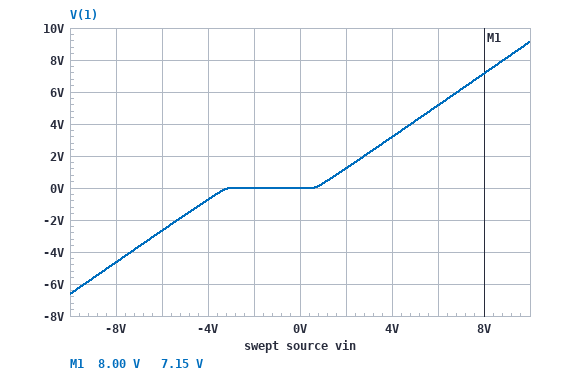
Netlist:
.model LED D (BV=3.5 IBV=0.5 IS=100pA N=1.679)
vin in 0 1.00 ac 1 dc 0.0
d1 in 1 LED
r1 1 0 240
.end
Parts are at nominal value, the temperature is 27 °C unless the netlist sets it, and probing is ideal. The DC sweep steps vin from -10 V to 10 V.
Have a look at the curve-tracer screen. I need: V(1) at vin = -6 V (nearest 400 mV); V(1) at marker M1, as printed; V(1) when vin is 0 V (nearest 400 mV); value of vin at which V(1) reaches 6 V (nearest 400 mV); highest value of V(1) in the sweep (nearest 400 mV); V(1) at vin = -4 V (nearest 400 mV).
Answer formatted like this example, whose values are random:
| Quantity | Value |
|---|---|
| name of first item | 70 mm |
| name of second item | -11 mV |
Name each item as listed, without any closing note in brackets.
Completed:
| Quantity | Value |
|---|---|
| V(1) at vin = -6 V | -2.8 V |
| V(1) at marker M1, as printed | 7.15 V |
| V(1) when vin is 0 V | 0 V |
| value of vin at which V(1) reaches 6 V | 6.8 V |
| highest value of V(1) in the sweep | 9.2 V |
| V(1) at vin = -4 V | -800 mV |
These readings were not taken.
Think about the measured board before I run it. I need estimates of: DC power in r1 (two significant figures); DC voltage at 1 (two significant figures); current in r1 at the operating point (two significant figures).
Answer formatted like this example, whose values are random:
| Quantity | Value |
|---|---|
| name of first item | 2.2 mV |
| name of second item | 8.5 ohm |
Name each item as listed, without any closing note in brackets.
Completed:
| Quantity | Value |
|---|---|
| DC power in r1 | 350 µW |
| DC voltage at 1 | 290 mV |
| current in r1 at the operating point | 1.2 mA |
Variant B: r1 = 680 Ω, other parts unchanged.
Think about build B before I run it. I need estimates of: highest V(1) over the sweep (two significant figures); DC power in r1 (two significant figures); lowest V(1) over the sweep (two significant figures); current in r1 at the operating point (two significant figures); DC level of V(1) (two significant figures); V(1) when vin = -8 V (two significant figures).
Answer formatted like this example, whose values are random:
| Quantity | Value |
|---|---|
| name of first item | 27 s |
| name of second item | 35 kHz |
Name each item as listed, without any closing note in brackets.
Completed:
| Quantity | Value |
|---|---|
| highest V(1) over the sweep | 9.2 V |
| DC power in r1 | 160 µW |
| lowest V(1) over the sweep | -6.7 V |
| current in r1 at the operating point | 490 µA |
| DC level of V(1) | 330 mV |
| V(1) when vin = -8 V | -4.7 V |
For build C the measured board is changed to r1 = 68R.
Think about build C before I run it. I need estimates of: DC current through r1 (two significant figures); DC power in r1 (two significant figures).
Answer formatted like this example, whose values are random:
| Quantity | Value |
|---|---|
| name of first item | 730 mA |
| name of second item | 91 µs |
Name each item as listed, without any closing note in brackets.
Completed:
| Quantity | Value |
|---|---|
| DC current through r1 | 3.6 mA |
| DC power in r1 | 880 µW |
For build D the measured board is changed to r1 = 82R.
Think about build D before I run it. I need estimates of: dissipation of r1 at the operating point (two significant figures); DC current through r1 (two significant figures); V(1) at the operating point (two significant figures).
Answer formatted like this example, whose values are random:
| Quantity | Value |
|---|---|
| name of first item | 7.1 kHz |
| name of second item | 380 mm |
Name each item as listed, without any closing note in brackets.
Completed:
| Quantity | Value |
|---|---|
| dissipation of r1 at the operating point | 770 µW |
| DC current through r1 | 3.1 mA |
| V(1) at the operating point | 250 mV |
